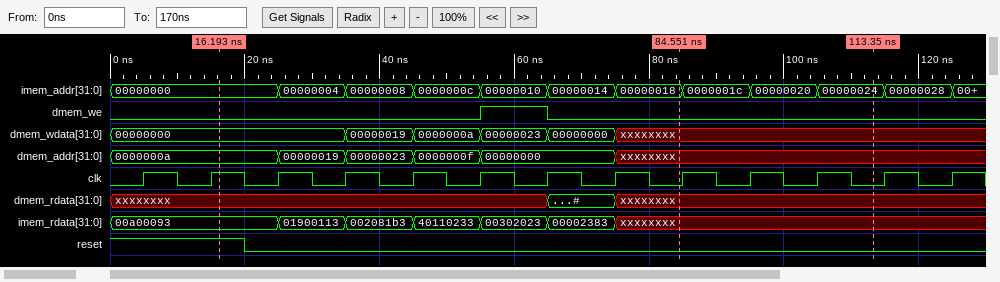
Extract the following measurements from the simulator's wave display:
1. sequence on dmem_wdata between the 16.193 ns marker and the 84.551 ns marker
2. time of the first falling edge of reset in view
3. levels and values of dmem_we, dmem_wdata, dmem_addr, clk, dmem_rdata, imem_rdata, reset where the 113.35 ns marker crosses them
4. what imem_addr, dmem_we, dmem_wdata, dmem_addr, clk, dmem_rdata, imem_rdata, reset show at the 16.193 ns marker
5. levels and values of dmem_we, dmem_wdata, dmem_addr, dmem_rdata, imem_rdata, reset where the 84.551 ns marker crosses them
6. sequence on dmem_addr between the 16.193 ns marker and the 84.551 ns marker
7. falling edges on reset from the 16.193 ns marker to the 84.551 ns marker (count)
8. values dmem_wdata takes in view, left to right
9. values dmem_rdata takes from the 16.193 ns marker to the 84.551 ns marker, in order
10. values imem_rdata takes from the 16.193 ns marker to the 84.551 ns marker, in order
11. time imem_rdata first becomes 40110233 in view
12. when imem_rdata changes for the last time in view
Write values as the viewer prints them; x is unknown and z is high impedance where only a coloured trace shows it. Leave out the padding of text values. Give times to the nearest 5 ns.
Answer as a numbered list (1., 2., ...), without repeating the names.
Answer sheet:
1. 00000000, 00000019, 0000000a, 00000023, 00000000, xxxxxxxx
2. 20 ns
3. dmem_we=0, dmem_wdata=xxxxxxxx, dmem_addr=xxxxxxxx, clk=0, dmem_rdata=xxxxxxxx, imem_rdata=xxxxxxxx, reset=0
4. imem_addr=00000000, dmem_we=0, dmem_wdata=00000000, dmem_addr=0000000a, clk=1, dmem_rdata=xxxxxxxx, imem_rdata=00a00093, reset=1
5. dmem_we=0, dmem_wdata=xxxxxxxx, dmem_addr=xxxxxxxx, dmem_rdata=xxxxxxxx, imem_rdata=xxxxxxxx, reset=0
6. 0000000a, 00000019, 00000023, 0000000f, 00000000, xxxxxxxx
7. 1
8. 00000000, 00000019, 0000000a, 00000023, 00000000, xxxxxxxx
9. xxxxxxxx, #, xxxxxxxx
10. 00a00093, 01900113, 002081b3, 40110233, 00302023, 00002383, xxxxxxxx
11. 45 ns
12. 75 ns
